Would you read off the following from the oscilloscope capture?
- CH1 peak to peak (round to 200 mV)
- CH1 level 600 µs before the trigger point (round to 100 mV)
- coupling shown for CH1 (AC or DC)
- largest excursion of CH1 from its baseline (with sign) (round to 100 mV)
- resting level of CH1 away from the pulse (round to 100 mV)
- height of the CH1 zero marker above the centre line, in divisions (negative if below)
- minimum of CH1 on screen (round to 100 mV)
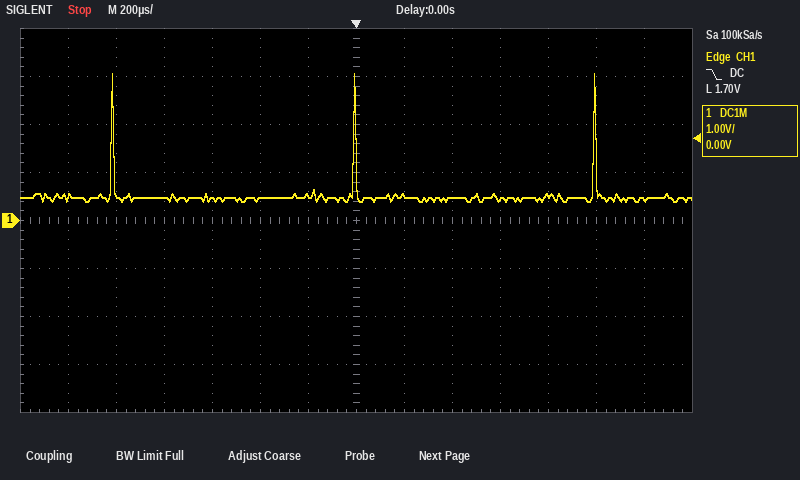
2.6 V
500 mV
DC
+2.6 V
500 mV
0.0 div
400 mV
